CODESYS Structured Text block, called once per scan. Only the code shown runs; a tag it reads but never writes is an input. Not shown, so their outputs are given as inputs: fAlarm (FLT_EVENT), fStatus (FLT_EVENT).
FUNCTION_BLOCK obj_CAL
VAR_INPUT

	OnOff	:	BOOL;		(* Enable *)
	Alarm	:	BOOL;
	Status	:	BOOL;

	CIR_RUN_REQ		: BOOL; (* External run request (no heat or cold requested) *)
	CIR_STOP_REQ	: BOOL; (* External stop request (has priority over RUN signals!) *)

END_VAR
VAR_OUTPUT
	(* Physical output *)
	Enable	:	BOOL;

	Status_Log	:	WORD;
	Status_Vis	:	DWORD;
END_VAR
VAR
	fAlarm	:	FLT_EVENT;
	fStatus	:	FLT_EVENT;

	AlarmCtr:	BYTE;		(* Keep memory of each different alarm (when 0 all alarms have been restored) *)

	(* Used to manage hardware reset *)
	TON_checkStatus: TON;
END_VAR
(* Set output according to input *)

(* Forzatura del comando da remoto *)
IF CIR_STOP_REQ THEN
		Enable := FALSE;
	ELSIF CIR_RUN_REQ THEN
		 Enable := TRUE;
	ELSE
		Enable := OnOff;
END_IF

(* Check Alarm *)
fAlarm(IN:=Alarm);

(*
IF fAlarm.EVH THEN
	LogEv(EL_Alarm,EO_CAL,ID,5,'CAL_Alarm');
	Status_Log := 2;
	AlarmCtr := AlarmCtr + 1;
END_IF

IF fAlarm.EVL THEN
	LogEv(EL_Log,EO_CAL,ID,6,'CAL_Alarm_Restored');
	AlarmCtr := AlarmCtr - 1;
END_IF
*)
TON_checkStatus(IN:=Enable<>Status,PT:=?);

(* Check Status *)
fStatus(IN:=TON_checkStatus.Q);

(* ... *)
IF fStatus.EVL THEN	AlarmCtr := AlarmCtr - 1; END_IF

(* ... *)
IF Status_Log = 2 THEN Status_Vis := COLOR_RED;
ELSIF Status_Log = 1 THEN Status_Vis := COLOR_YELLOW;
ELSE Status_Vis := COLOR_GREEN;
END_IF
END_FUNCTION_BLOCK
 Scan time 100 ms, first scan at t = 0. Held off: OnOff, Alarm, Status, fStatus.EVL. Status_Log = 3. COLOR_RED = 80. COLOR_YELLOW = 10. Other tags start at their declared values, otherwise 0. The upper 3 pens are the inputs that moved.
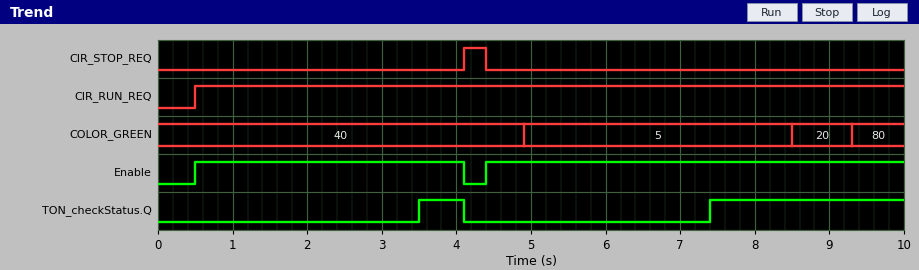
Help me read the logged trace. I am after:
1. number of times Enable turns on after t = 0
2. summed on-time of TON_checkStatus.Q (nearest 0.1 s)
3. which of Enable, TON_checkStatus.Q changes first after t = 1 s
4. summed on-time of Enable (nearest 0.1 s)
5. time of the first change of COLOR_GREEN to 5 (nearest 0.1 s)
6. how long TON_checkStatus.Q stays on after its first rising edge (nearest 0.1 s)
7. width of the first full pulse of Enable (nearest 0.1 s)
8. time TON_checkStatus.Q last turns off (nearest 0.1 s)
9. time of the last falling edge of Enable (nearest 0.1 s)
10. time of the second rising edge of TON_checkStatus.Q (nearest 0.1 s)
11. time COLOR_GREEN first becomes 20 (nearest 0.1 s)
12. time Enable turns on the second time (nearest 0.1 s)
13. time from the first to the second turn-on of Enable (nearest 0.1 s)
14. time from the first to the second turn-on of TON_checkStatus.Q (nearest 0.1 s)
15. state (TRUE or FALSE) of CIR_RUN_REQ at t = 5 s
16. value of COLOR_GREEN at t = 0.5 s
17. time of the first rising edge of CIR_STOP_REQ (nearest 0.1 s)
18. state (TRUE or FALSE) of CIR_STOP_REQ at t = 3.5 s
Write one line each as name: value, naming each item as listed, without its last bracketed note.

number of times Enable turns on after t = 0: 2
summed on-time of TON_checkStatus.Q: 3.2 s
which of Enable, TON_checkStatus.Q changes first after t = 1 s: TON_checkStatus.Q
summed on-time of Enable: 9.2 s
time of the first change of COLOR_GREEN to 5: 4.9 s
how long TON_checkStatus.Q stays on after its first rising edge: 0.6 s
width of the first full pulse of Enable: 3.6 s
time TON_checkStatus.Q last turns off: 4.1 s
time of the last falling edge of Enable: 4.1 s
time of the second rising edge of TON_checkStatus.Q: 7.4 s
time COLOR_GREEN first becomes 20: 8.5 s
time Enable turns on the second time: 4.4 s
time from the first to the second turn-on of Enable: 3.9 s
time from the first to the second turn-on of TON_checkStatus.Q: 3.9 s
state (TRUE or FALSE) of CIR_RUN_REQ at t = 5 s: TRUE
value of COLOR_GREEN at t = 0.5 s: 40
time of the first rising edge of CIR_STOP_REQ: 4.1 s
state (TRUE or FALSE) of CIR_STOP_REQ at t = 3.5 s: FALSE
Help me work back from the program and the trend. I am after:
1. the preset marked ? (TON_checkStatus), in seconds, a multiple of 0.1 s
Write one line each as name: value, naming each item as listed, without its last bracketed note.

the preset marked ? (TON_checkStatus), in seconds, a multiple of 0.1 s: 3.0 s
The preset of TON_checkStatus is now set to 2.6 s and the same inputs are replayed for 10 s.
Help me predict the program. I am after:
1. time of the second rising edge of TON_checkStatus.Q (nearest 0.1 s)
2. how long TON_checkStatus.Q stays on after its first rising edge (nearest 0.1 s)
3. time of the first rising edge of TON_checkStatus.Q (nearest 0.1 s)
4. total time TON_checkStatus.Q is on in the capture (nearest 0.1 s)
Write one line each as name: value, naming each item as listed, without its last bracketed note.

time of the second rising edge of TON_checkStatus.Q: 7.0 s
how long TON_checkStatus.Q stays on after its first rising edge: 1.0 s
time of the first rising edge of TON_checkStatus.Q: 3.1 s
total time TON_checkStatus.Q is on in the capture: 4.0 s
